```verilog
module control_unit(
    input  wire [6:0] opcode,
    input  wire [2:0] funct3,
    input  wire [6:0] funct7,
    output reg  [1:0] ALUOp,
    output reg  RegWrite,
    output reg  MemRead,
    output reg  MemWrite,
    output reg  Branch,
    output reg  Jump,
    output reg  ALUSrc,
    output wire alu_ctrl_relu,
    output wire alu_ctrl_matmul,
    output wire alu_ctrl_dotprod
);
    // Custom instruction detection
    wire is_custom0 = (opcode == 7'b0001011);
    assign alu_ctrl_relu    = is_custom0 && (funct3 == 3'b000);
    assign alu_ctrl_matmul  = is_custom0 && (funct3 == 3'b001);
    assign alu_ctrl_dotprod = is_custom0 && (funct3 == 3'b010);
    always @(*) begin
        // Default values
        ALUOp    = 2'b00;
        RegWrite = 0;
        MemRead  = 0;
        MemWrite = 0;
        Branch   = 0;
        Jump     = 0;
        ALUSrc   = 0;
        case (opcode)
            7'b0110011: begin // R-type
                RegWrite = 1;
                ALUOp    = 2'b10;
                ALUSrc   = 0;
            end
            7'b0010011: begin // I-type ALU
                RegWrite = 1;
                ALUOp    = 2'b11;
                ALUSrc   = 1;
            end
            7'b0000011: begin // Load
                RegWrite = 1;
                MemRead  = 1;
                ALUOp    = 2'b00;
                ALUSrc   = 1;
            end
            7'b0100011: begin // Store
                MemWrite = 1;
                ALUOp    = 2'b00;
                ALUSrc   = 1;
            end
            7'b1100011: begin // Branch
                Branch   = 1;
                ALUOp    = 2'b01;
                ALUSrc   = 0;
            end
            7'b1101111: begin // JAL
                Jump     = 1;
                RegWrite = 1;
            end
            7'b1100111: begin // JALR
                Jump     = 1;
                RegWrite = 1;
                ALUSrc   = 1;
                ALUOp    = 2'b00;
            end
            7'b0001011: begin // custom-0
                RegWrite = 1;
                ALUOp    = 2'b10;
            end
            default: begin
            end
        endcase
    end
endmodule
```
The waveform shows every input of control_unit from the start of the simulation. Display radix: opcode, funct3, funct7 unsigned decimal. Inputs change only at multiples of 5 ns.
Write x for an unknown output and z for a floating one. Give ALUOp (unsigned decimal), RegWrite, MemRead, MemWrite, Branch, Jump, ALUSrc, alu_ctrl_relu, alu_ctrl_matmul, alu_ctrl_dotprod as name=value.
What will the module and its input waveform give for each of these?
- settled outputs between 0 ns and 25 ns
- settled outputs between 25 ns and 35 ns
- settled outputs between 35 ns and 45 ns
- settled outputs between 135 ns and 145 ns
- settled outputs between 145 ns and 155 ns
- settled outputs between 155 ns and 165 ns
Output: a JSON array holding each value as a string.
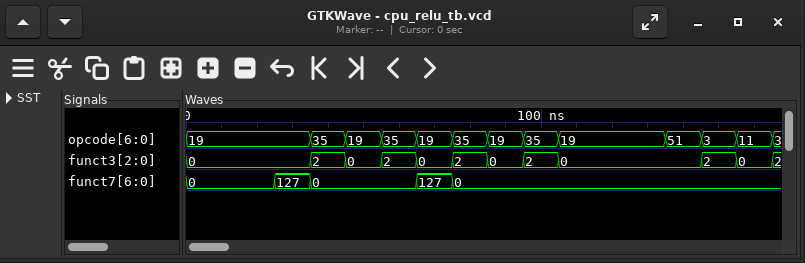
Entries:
["ALUOp=3, RegWrite=1, MemRead=0, MemWrite=0, Branch=0, Jump=0, ALUSrc=1, alu_ctrl_relu=0, alu_ctrl_matmul=0, alu_ctrl_dotprod=0", "ALUOp=3, RegWrite=1, MemRead=0, MemWrite=0, Branch=0, Jump=0, ALUSrc=1, alu_ctrl_relu=0, alu_ctrl_matmul=0, alu_ctrl_dotprod=0", "ALUOp=0, RegWrite=0, MemRead=0, MemWrite=1, Branch=0, Jump=0, ALUSrc=1, alu_ctrl_relu=0, alu_ctrl_matmul=0, alu_ctrl_dotprod=0", "ALUOp=2, RegWrite=1, MemRead=0, MemWrite=0, Branch=0, Jump=0, ALUSrc=0, alu_ctrl_relu=0, alu_ctrl_matmul=0, alu_ctrl_dotprod=0", "ALUOp=0, RegWrite=1, MemRead=1, MemWrite=0, Branch=0, Jump=0, ALUSrc=1, alu_ctrl_relu=0, alu_ctrl_matmul=0, alu_ctrl_dotprod=0", "ALUOp=2, RegWrite=1, MemRead=0, MemWrite=0, Branch=0, Jump=0, ALUSrc=0, alu_ctrl_relu=1, alu_ctrl_matmul=0, alu_ctrl_dotprod=0"]
